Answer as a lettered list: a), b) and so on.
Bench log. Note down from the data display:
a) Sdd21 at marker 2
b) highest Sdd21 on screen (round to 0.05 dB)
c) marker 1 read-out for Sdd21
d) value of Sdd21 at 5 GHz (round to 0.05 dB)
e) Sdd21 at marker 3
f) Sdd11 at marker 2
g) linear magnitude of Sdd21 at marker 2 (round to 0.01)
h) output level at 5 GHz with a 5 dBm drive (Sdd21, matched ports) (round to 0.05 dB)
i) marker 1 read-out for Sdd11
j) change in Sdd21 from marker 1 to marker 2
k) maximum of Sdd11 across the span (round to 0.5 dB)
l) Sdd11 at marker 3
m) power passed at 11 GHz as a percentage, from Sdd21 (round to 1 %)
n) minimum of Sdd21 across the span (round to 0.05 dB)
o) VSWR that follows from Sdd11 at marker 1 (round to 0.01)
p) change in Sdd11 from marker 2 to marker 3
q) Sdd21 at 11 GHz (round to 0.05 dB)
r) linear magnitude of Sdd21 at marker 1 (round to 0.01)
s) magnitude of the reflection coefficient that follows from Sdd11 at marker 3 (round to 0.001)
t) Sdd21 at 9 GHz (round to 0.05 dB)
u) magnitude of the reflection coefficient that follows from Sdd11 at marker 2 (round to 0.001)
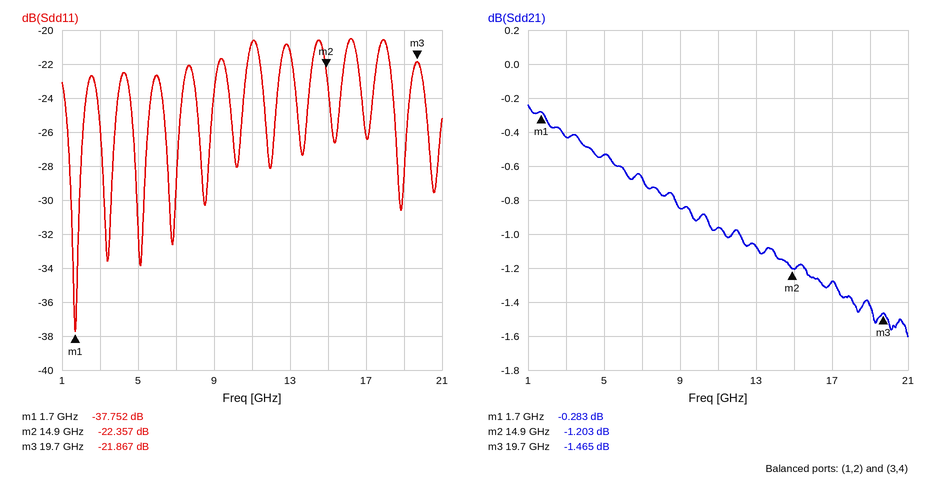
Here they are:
a) -1.203 dB
b) -0.25 dB
c) -0.283 dB
d) -0.55 dB
e) -1.465 dB
f) -22.357 dB
g) 0.87
h) 4.45 dBm
i) -37.752 dB
j) -0.920 dB
k) -20.5 dB
l) -21.867 dB
m) 80 %
n) -1.60 dB
o) 1.03
p) 0.490 dB
q) -0.95 dB
r) 0.97
s) 0.081
t) -0.85 dB
u) 0.076
